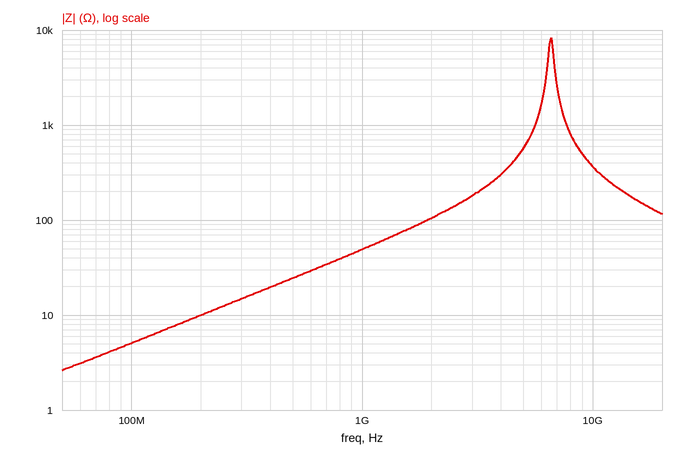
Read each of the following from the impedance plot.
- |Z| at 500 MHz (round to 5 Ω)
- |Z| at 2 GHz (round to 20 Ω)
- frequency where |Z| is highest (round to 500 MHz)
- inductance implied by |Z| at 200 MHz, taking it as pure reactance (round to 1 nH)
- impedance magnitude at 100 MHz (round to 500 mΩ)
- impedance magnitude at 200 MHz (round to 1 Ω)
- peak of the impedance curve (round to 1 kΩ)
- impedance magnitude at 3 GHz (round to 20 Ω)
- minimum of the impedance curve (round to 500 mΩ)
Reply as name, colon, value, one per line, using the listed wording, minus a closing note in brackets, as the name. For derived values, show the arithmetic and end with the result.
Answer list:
|Z| at 500 MHz: 25 Ω
|Z| at 2 GHz: 100 Ω
frequency where |Z| is highest: 6.5 GHz
inductance implied by |Z| at 200 MHz, taking it as pure reactance: L = 10 Ω/(2π × 200 MHz) ≈ 8 nH
impedance magnitude at 100 MHz: 5.0 Ω
impedance magnitude at 200 MHz: 10 Ω
peak of the impedance curve: 8 kΩ
impedance magnitude at 3 GHz: 180 Ω
minimum of the impedance curve: 2.5 Ω
